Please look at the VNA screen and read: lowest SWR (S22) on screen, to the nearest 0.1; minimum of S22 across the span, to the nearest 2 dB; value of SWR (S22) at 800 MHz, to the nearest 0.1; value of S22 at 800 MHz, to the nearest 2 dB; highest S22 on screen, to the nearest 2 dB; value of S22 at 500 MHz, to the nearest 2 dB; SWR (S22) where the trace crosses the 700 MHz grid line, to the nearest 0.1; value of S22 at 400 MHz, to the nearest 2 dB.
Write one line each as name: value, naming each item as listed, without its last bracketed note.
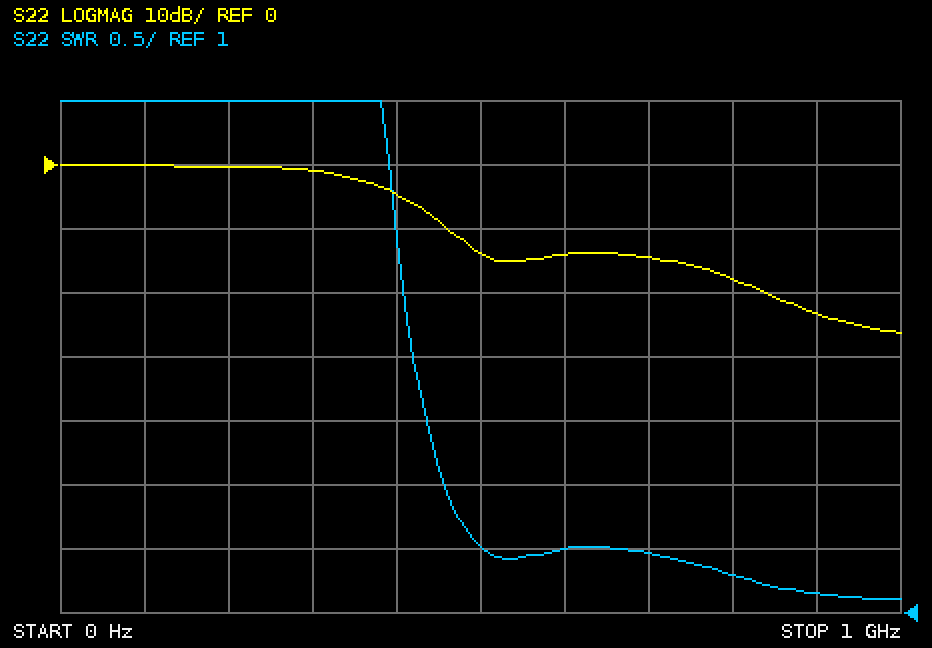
lowest SWR (S22) on screen, to the nearest 0.1: 1.1
minimum of S22 across the span, to the nearest 2 dB: -26 dB
value of SWR (S22) at 800 MHz, to the nearest 0.1: 1.3
value of S22 at 800 MHz, to the nearest 2 dB: -18 dB
highest S22 on screen, to the nearest 2 dB: 0 dB
value of S22 at 500 MHz, to the nearest 2 dB: -14 dB
SWR (S22) where the trace crosses the 700 MHz grid line, to the nearest 0.1: 1.5
value of S22 at 400 MHz, to the nearest 2 dB: -4 dB
